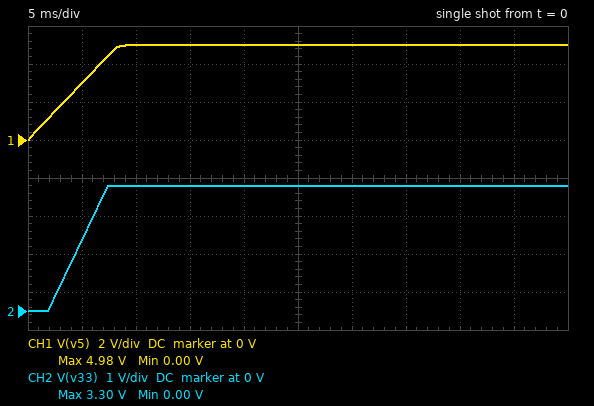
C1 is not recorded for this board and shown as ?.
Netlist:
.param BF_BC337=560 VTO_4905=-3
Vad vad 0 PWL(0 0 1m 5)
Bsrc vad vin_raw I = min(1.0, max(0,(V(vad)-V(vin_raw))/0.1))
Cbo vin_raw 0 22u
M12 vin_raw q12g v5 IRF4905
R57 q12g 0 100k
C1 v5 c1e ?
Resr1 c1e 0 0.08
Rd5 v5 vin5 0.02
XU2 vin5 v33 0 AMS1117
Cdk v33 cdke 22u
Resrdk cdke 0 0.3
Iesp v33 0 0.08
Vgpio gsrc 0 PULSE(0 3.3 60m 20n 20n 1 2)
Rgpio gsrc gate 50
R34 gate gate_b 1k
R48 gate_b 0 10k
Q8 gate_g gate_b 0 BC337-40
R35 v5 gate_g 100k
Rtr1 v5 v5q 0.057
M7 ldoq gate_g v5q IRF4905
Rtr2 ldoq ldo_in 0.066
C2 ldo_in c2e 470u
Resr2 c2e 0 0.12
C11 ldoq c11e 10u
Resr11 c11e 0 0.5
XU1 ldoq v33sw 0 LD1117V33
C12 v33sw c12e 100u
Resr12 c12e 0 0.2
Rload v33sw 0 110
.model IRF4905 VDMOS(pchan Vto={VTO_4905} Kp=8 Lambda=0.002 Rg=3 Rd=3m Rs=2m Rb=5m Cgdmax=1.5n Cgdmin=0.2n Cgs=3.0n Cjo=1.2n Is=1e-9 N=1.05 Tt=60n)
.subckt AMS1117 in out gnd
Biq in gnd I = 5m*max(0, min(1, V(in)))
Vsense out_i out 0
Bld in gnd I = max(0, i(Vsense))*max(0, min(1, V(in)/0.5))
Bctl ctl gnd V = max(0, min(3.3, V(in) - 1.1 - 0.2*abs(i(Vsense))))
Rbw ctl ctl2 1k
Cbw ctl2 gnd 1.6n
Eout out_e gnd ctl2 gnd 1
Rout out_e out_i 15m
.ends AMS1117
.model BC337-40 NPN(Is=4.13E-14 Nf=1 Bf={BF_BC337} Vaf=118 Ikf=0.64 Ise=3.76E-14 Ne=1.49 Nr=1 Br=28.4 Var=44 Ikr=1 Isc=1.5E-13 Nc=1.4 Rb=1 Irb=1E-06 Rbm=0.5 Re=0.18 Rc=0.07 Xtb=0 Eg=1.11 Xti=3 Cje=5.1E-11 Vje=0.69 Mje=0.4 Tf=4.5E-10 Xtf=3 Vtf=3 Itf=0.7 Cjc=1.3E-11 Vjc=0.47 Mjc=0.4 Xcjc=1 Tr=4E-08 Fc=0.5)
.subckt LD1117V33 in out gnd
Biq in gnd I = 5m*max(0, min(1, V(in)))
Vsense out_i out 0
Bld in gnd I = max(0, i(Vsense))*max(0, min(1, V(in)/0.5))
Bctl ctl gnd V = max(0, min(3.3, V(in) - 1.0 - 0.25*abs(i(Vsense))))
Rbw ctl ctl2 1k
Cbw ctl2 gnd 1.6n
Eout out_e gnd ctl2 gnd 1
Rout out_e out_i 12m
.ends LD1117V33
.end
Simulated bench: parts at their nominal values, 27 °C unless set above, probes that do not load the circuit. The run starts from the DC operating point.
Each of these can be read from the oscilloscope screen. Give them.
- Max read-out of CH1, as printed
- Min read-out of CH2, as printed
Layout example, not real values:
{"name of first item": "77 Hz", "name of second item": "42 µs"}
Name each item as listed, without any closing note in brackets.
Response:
{"Max read-out of CH1, as printed": "4.98 V", "Min read-out of CH2, as printed": "0.00 V"}
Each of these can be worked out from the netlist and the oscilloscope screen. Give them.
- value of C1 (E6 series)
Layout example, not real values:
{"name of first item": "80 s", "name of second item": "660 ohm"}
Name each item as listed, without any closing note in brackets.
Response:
{"value of C1": "1.5 mF"}
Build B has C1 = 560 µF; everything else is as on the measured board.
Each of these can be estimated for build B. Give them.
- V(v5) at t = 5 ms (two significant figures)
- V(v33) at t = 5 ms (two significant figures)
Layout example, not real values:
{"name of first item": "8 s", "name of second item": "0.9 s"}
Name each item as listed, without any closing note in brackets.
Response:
{"V(v5) at t = 5 ms": "5.0 V", "V(v33) at t = 5 ms": "3.3 V"}
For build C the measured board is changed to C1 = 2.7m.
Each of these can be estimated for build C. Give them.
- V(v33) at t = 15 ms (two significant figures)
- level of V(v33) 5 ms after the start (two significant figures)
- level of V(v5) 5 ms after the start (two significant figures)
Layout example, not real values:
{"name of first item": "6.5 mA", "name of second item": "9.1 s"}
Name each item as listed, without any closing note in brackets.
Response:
{"V(v33) at t = 15 ms": "3.3 V", "level of V(v33) 5 ms after the start": "600 mV", "level of V(v5) 5 ms after the start": "1.7 V"}
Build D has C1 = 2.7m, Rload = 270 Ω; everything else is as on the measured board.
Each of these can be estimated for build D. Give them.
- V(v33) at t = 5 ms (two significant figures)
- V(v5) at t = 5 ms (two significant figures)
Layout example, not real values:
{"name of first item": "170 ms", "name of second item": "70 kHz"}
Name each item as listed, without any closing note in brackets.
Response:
{"V(v33) at t = 5 ms": "600 mV", "V(v5) at t = 5 ms": "1.7 V"}
